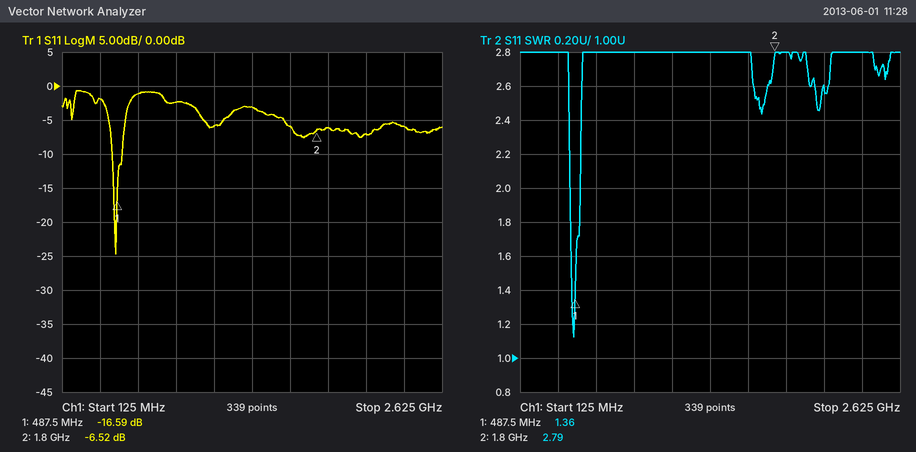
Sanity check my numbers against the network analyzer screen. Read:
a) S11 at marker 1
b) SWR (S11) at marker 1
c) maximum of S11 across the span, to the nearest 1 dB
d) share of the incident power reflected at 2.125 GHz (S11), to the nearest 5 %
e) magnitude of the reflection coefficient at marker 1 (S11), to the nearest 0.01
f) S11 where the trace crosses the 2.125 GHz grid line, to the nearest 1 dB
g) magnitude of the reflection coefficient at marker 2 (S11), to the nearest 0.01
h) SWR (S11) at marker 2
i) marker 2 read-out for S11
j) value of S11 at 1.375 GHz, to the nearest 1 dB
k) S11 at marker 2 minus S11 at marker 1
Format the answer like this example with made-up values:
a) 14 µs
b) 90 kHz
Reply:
a) -16.59 dB
b) 1.36
c) -1 dB
d) 20 %
e) 0.15
f) -7 dB
g) 0.47
h) 2.79
i) -6.52 dB
j) -3 dB
k) 10.07 dB
